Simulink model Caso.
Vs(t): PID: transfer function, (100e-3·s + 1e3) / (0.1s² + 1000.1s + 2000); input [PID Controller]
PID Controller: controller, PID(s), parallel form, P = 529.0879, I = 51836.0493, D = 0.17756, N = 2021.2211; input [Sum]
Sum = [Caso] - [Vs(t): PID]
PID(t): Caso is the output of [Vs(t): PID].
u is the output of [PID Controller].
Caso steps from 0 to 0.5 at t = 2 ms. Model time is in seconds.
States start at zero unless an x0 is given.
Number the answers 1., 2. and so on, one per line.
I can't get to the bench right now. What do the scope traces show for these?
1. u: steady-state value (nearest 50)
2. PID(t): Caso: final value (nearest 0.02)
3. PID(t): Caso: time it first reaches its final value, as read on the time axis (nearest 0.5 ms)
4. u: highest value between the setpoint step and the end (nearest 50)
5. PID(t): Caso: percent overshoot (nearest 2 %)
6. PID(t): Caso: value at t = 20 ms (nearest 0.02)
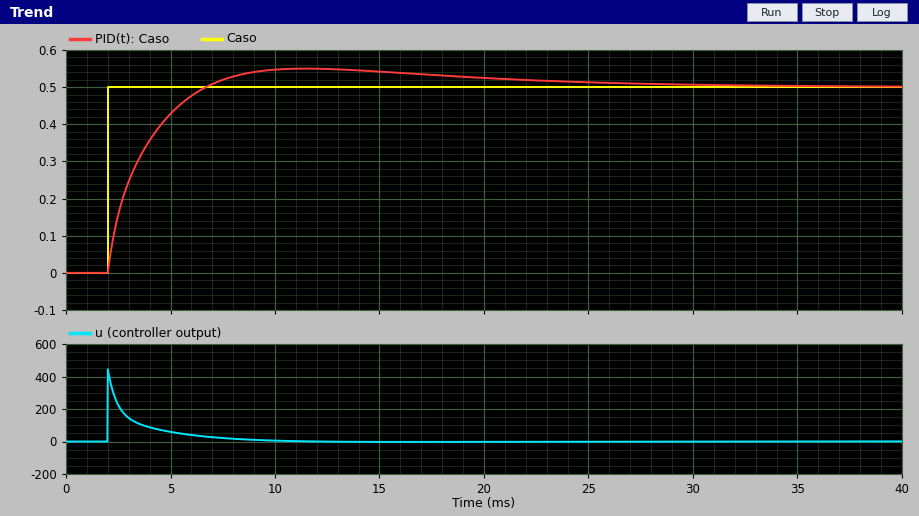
1. 0
2. 0.50
3. 6.5 ms
4. 450
5. 10 %
6. 0.52
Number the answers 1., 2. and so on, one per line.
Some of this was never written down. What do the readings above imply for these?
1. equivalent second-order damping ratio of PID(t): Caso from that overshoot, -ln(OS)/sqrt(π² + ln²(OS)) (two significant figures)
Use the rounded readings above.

1. 0.59
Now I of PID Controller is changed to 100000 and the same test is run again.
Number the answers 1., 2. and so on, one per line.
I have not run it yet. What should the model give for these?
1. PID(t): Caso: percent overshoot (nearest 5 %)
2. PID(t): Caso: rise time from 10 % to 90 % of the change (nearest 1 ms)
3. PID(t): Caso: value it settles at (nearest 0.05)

1. 15 %
2. 3 ms
3. 0.50
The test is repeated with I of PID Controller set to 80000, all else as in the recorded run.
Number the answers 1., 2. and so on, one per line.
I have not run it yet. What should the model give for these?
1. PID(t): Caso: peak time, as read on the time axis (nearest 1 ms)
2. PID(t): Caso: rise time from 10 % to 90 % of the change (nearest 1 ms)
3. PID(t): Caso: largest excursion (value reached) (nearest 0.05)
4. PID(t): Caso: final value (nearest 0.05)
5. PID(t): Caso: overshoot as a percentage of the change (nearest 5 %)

1. 10 ms
2. 3 ms
3. 0.55
4. 0.50
5. 15 %
